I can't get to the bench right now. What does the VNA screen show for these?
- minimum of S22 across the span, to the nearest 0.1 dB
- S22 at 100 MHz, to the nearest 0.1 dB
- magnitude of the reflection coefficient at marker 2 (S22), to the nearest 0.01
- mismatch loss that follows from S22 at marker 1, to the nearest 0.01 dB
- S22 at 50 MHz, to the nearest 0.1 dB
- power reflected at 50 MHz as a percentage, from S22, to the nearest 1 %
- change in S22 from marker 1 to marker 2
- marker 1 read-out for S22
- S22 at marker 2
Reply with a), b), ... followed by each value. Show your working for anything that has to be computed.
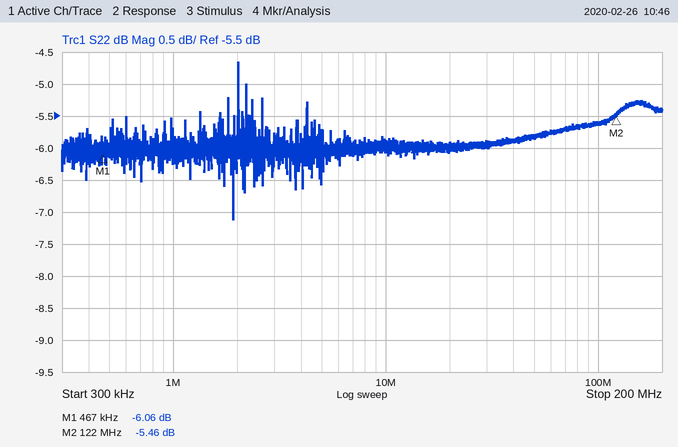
a) -7.1 dB
b) -5.6 dB
c) 10^(-5.46/20) ≈ 0.53
d) −10 log10(1 − 10^(-6.06/10)) ≈ 1.24 dB
e) -5.8 dB
f) 10^(-5.8/10) ≈ 26 %
g) -5.46 − (-6.06) = 0.60 dB
h) -6.06 dB
i) -5.46 dB
